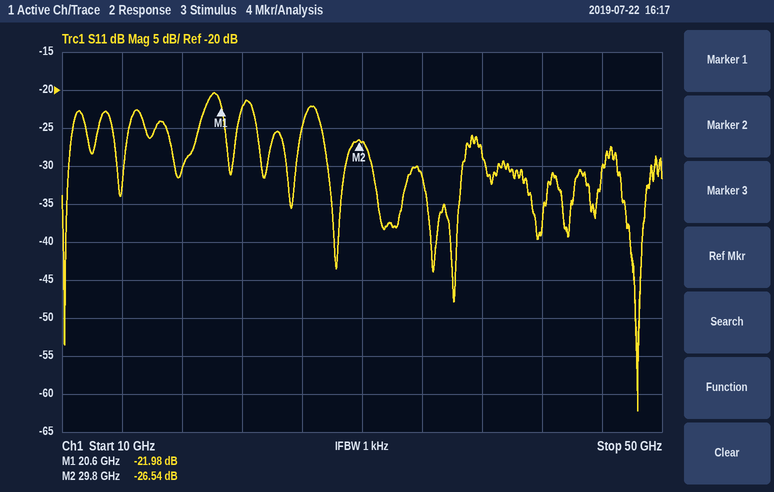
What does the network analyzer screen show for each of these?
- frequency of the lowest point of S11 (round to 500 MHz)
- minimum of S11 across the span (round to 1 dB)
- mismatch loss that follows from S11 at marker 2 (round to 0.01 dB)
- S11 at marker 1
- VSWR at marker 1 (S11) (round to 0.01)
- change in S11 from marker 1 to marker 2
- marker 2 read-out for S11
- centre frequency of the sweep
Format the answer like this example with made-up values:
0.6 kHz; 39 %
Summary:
48.5 GHz; -62 dB; 0.01 dB; -21.98 dB; 1.17; -4.56 dB; -26.54 dB; 30 GHz
